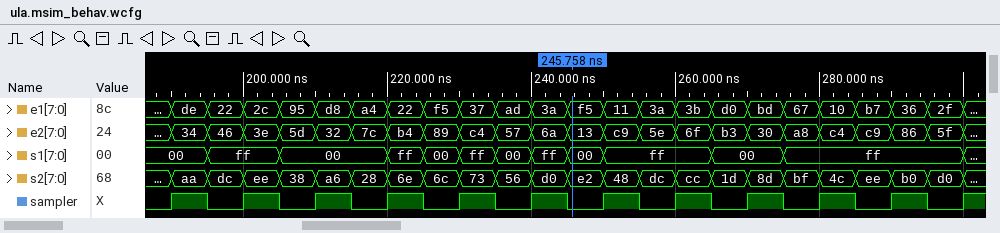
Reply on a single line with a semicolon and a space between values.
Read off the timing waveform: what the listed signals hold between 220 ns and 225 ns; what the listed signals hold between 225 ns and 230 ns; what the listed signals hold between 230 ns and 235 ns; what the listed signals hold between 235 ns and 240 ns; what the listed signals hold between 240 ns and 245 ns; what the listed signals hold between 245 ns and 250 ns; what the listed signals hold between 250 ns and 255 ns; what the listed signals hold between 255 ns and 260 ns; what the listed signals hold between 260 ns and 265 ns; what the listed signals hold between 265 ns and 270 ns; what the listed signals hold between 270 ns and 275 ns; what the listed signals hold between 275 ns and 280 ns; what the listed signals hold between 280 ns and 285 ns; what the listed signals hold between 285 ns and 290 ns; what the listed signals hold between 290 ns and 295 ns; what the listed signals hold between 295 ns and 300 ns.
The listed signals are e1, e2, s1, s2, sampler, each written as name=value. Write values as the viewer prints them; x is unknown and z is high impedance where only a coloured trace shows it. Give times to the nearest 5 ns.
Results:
e1=22, e2=b4, s1=ff, s2=6e, sampler=1; e1=f5, e2=89, s1=00, s2=6c, sampler=0; e1=37, e2=c4, s1=ff, s2=73, sampler=1; e1=ad, e2=57, s1=00, s2=56, sampler=0; e1=3a, e2=6a, s1=ff, s2=d0, sampler=1; e1=f5, e2=13, s1=00, s2=e2, sampler=0; e1=11, e2=c9, s1=ff, s2=48, sampler=1; e1=3a, e2=5e, s1=ff, s2=dc, sampler=0; e1=3b, e2=6f, s1=ff, s2=cc, sampler=1; e1=d0, e2=b3, s1=00, s2=1d, sampler=0; e1=bd, e2=30, s1=00, s2=8d, sampler=1; e1=67, e2=a8, s1=ff, s2=bf, sampler=0; e1=10, e2=c4, s1=ff, s2=4c, sampler=1; e1=b7, e2=c9, s1=ff, s2=ee, sampler=0; e1=36, e2=86, s1=ff, s2=b0, sampler=1; e1=2f, e2=5f, s1=ff, s2=d0, sampler=0
